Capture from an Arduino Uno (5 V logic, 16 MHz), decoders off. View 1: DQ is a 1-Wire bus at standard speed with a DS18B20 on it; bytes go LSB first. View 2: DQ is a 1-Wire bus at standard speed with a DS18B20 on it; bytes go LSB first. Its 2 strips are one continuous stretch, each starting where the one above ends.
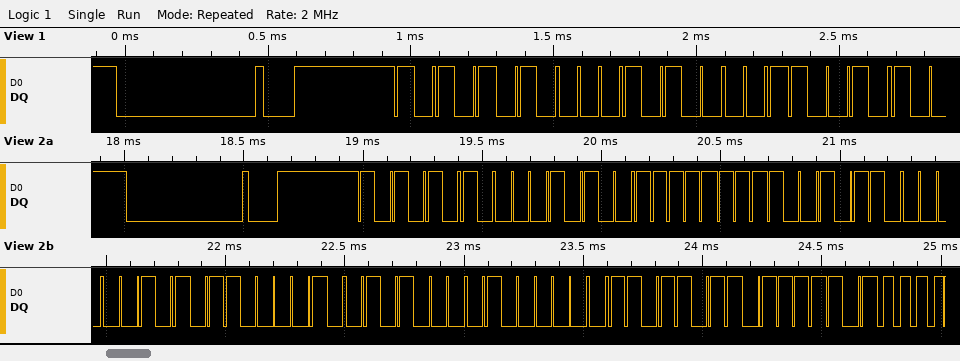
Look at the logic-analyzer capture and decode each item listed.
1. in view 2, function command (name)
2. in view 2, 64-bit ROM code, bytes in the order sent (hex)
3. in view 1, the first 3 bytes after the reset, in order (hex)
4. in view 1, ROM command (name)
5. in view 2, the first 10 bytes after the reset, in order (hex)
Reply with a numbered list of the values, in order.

1. Read Scratchpad
2. 28 FF 69 A0 86 14 02 DB
3. 55 28 4C
4. Match ROM
5. 55 28 FF 69 A0 86 14 02 DB BE
